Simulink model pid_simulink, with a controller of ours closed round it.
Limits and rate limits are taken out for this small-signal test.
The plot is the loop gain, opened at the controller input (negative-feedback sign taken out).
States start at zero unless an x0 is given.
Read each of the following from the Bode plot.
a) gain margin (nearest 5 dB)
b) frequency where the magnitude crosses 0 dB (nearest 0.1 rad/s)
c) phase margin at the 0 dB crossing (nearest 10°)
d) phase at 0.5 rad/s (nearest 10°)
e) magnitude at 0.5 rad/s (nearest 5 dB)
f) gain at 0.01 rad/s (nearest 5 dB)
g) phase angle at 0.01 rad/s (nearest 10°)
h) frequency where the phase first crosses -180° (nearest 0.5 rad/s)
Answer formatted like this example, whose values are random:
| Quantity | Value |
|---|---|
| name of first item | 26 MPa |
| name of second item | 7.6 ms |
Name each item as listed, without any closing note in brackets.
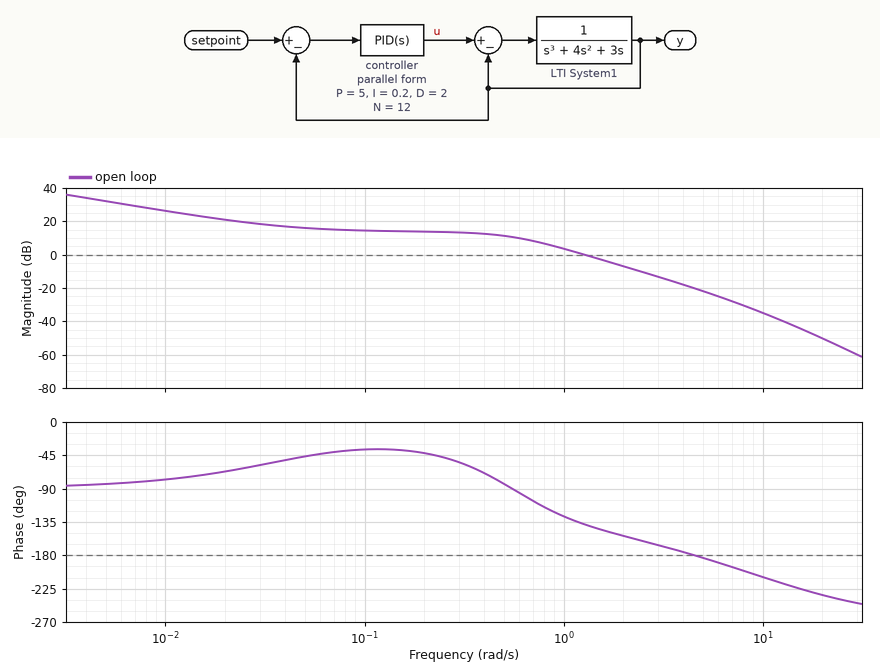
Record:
| Quantity | Value |
|---|---|
| gain margin | 20 dB |
| frequency where the magnitude crosses 0 dB | 1.3 rad/s |
| phase margin at the 0 dB crossing | 40° |
| phase at 0.5 rad/s | -80° |
| magnitude at 0.5 rad/s | 10 dB |
| gain at 0.01 rad/s | 25 dB |
| phase angle at 0.01 rad/s | -80° |
| frequency where the phase first crosses -180° | 4.5 rad/s |
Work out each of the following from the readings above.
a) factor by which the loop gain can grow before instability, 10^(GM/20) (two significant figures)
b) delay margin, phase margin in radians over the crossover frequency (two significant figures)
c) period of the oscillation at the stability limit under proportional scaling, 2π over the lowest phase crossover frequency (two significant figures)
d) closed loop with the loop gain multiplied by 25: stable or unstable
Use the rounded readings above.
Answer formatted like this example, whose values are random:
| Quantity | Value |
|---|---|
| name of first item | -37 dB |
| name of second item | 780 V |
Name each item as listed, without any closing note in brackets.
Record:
| Quantity | Value |
|---|---|
| factor by which the loop gain can grow before instability, 10^(GM/20) | 10 |
| delay margin, phase margin in radians over the crossover frequency | 0.54 s |
| period of the oscillation at the stability limit under proportional scaling, 2π over the lowest phase crossover frequency | 1.4 s |
| closed loop with the loop gain multiplied by 25: stable or unstable | unstable |
